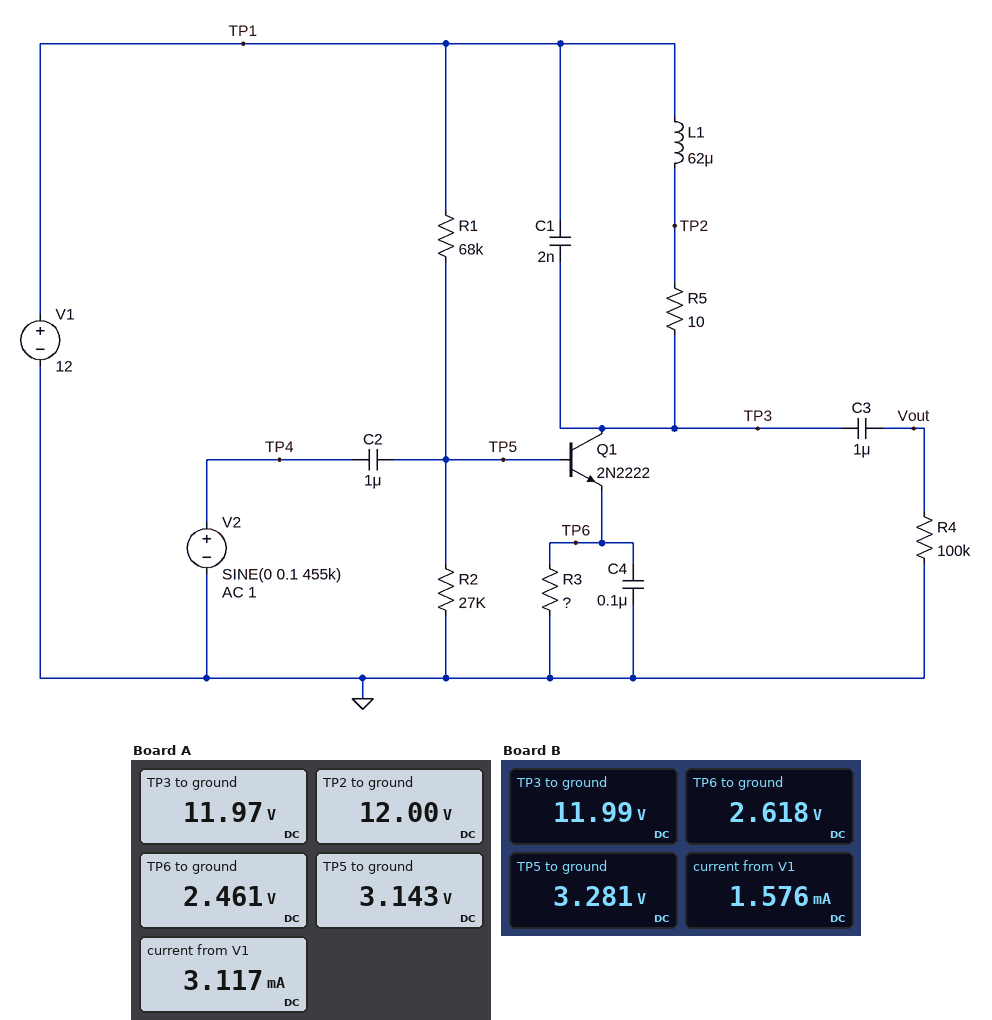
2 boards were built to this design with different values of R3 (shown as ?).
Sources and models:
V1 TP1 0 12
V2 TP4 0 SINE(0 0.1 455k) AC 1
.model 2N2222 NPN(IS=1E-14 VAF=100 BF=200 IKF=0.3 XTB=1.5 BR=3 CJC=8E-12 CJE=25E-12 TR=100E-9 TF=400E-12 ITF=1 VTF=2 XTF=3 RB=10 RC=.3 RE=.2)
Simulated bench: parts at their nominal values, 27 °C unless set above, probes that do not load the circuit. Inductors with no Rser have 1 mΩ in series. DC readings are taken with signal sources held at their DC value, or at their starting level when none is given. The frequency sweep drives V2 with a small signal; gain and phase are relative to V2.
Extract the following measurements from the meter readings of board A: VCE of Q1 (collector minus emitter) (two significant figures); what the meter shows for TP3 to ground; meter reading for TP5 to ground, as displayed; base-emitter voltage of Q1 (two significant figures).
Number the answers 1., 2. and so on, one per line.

1. 9.5 V
2. 11.97 V
3. 3.143 V
4. 680 mV
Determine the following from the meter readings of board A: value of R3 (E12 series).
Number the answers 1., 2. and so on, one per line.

1. 820 Ω
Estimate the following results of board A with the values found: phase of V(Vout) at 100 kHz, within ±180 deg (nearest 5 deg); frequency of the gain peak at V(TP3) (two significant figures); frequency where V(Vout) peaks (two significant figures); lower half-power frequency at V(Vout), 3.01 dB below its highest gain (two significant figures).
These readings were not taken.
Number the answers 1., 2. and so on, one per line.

1. -45 deg
2. 450 kHz
3. 450 kHz
4. 440 kHz
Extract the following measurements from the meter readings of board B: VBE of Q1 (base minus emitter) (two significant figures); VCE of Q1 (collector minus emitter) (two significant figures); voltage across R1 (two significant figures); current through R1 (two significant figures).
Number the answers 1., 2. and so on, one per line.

1. 660 mV
2. 9.4 V
3. 8.7 V
4. 130 µA
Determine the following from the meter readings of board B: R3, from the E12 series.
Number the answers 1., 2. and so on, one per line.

1. 1.8 kΩ
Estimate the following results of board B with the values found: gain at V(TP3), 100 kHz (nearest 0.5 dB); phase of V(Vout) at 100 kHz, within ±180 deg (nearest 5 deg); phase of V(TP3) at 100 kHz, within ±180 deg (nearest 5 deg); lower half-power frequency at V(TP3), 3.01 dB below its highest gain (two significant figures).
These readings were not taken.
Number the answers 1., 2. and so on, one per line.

1. 5.0 dB
2. -65 deg
3. -65 deg
4. 440 kHz
